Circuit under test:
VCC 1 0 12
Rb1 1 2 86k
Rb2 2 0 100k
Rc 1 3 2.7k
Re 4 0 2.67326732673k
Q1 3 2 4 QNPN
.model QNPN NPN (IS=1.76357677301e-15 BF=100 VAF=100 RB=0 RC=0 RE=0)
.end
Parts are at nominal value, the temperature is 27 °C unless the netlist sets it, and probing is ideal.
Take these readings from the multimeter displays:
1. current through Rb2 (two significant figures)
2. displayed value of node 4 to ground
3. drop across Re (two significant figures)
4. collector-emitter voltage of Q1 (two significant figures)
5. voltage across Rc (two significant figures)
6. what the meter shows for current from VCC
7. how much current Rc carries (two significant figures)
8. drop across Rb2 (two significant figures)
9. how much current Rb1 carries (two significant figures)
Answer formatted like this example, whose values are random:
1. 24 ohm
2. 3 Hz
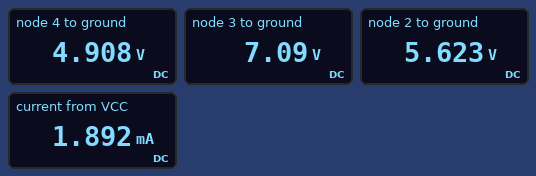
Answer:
1. 56 µA
2. 4.908 V
3. 4.9 V
4. 2.2 V
5. 4.9 V
6. 1.892 mA
7. 1.8 mA
8. 5.6 V
9. 74 µA
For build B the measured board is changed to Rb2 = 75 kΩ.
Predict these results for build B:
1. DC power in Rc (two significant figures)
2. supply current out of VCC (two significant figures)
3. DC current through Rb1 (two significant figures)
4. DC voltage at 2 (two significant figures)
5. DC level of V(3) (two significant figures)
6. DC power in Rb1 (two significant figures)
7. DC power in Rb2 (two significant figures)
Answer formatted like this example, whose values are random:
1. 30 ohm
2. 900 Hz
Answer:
1. 6.7 mW
2. 1.7 mA
3. 82 µA
4. 5.0 V
5. 7.7 V
6. 570 µW
7. 330 µW
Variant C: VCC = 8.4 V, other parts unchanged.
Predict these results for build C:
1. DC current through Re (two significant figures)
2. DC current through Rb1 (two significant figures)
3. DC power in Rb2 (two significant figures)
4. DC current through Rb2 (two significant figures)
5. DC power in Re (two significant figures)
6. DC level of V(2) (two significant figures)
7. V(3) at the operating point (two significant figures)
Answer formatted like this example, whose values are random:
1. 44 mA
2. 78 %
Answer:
1. 1.2 mA
2. 52 µA
3. 160 µW
4. 40 µA
5. 4.0 mW
6. 4.0 V
7. 5.1 V
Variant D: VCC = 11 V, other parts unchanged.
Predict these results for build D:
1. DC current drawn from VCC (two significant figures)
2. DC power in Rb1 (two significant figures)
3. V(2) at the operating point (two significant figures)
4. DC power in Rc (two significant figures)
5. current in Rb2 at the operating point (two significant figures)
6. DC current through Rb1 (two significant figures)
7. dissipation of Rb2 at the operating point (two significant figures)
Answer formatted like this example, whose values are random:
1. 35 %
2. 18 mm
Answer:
1. 1.7 mA
2. 400 µW
3. 5.2 V
4. 7.3 mW
5. 52 µA
6. 68 µA
7. 270 µW
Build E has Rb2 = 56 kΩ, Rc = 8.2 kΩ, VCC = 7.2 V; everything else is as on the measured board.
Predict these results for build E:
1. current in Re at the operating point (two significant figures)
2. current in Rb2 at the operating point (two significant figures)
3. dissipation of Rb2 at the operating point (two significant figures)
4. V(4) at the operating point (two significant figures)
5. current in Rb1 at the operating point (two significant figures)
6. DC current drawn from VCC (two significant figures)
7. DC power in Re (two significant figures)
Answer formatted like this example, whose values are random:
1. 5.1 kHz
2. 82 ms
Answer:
1. 660 µA
2. 44 µA
3. 110 µW
4. 1.8 V
5. 55 µA
6. 700 µA
7. 1.2 mW
